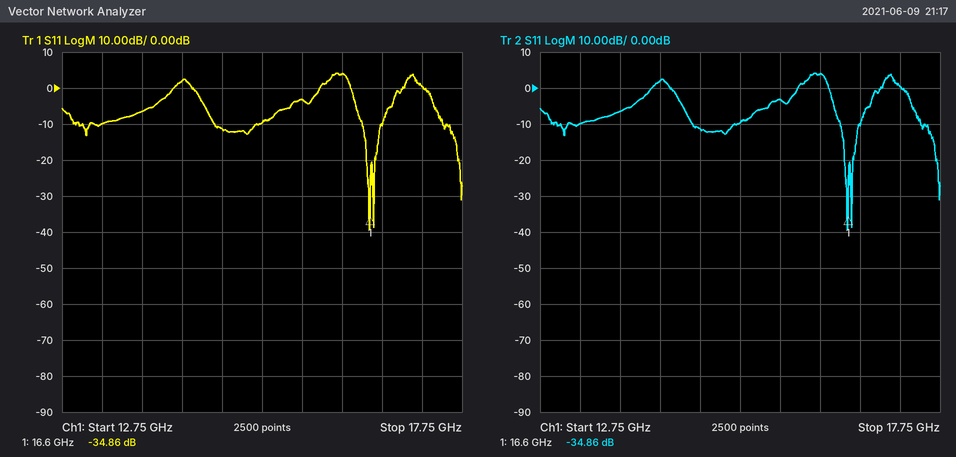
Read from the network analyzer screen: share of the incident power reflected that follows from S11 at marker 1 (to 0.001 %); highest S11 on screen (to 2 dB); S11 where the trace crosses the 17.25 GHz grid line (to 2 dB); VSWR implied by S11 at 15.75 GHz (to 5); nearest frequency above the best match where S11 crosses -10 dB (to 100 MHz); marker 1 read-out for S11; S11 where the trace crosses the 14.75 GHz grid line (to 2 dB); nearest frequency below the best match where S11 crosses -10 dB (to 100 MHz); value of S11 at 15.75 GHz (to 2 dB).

0.033 %
4 dB
0 dB
5
16.7 GHz
-34.86 dB
-12 dB
16.5 GHz
-4 dB
